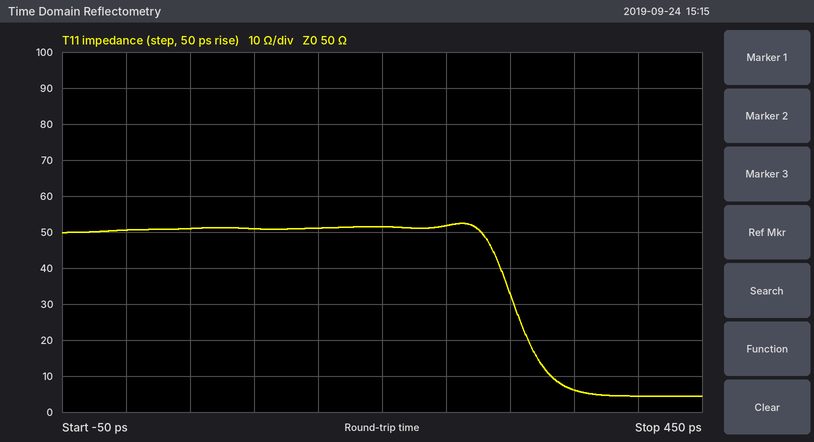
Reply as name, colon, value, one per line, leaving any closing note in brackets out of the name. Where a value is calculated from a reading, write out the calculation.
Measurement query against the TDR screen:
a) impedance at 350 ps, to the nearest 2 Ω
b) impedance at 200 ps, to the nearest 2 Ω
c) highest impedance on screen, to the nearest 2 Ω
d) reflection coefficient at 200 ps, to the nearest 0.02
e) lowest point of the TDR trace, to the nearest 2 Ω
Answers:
impedance at 350 ps, to the nearest 2 Ω: 6 Ω
impedance at 200 ps, to the nearest 2 Ω: 52 Ω
highest impedance on screen, to the nearest 2 Ω: 52 Ω
reflection coefficient at 200 ps, to the nearest 0.02: (52 − 50)/(52 + 50) ≈ +0.02
lowest point of the TDR trace, to the nearest 2 Ω: 4 Ω
